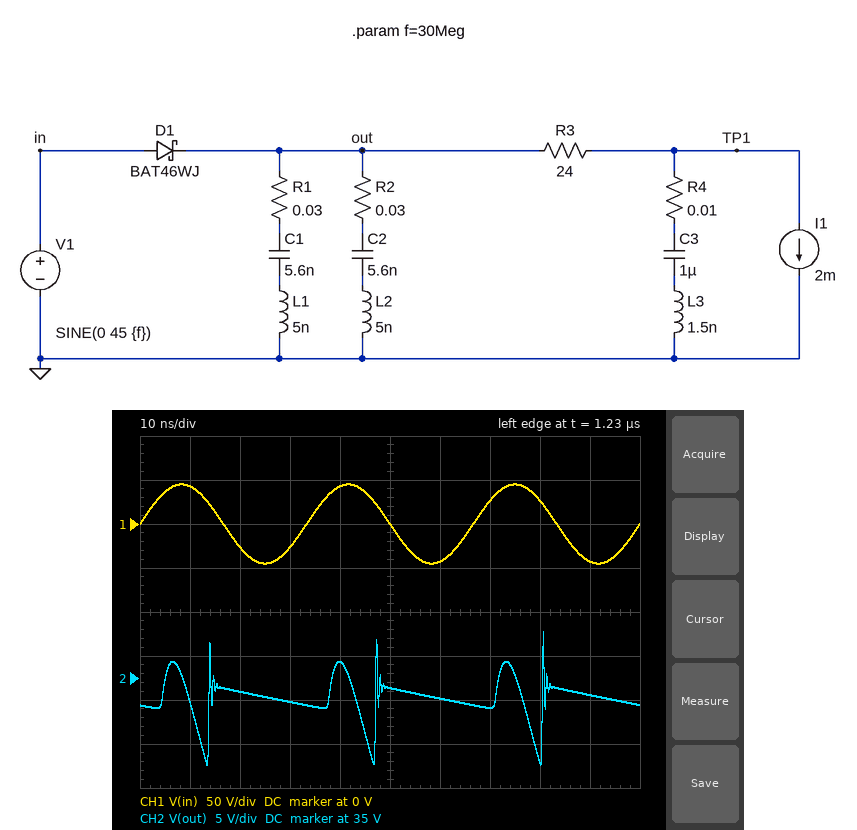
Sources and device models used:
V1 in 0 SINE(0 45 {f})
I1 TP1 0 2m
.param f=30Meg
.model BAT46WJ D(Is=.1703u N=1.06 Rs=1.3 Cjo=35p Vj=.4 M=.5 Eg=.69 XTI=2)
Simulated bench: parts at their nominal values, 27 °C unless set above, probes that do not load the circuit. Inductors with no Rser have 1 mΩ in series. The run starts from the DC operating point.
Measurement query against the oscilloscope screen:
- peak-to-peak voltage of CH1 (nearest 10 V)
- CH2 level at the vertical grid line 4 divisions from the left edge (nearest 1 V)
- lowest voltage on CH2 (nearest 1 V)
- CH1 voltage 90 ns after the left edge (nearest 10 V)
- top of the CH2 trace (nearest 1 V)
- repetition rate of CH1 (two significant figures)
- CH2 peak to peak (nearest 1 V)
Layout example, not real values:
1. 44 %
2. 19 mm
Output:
1. 90 V
2. 37 V
3. 25 V
4. -40 V
5. 40 V
6. 30 MHz
7. 15 V
